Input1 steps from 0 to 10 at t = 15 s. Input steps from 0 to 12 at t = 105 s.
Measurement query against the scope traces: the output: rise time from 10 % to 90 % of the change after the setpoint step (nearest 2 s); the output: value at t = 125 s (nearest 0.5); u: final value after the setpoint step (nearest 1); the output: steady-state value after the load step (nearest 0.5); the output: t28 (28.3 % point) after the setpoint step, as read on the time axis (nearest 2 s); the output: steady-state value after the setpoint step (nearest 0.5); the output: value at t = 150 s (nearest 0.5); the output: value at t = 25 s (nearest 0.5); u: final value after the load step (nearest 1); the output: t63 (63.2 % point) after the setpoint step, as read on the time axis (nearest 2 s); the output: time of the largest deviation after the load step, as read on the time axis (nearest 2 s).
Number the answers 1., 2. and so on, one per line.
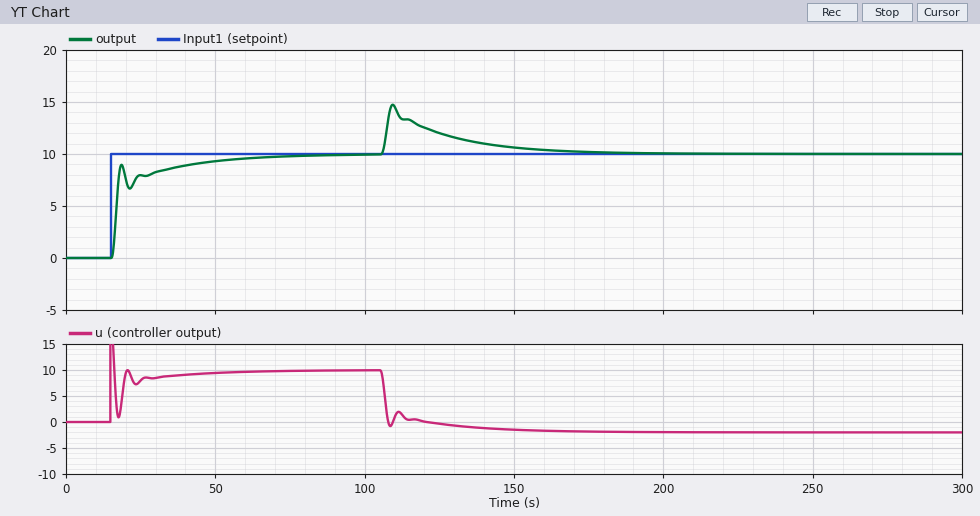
1. 26 s
2. 12.0
3. 10
4. 10.0
5. 16 s
6. 10.0
7. 10.5
8. 8.0
9. -2
10. 18 s
11. 110 s
